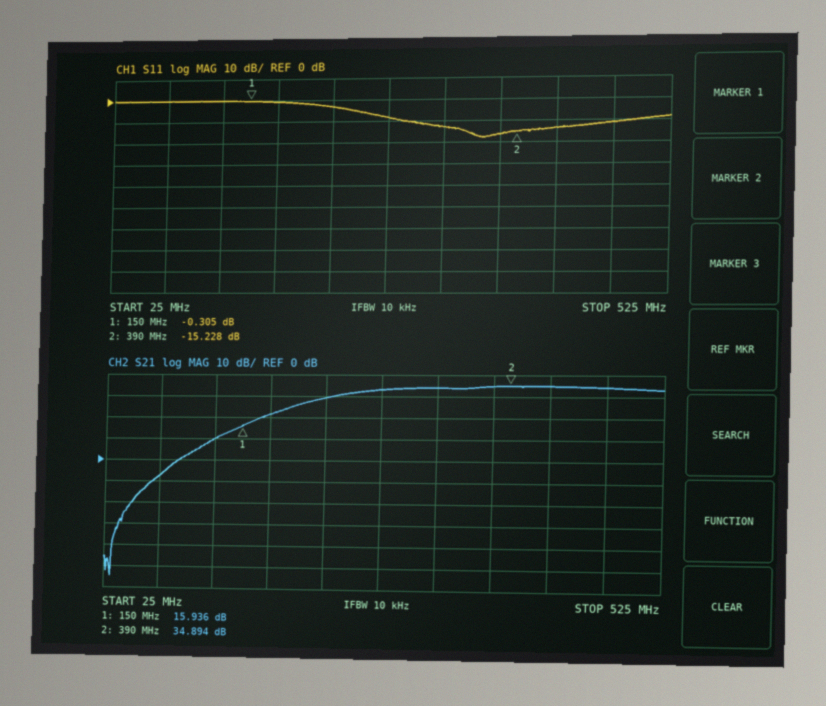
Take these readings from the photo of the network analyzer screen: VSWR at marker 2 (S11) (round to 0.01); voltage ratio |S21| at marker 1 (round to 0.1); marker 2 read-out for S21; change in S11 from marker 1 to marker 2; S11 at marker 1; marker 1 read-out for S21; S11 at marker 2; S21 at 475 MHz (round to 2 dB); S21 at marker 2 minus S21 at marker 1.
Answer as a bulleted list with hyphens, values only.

- 1.42
- 6.3
- 34.894 dB
- -14.923 dB
- -0.305 dB
- 15.936 dB
- -15.228 dB
- 34 dB
- 18.958 dB
